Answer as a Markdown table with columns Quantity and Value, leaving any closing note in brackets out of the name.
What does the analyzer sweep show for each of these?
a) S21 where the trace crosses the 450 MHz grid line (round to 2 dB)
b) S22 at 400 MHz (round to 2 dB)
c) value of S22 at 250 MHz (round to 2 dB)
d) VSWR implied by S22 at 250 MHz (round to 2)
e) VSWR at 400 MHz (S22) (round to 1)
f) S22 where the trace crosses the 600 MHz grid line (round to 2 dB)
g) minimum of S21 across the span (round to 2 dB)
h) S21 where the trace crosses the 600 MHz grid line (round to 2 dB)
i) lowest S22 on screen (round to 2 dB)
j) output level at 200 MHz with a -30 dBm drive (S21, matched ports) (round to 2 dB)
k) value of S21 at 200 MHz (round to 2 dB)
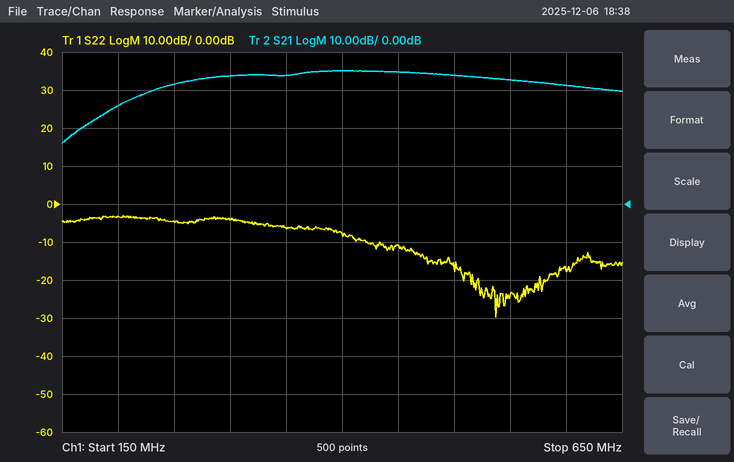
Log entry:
| Quantity | Value |
|---|---|
| S21 where the trace crosses the 450 MHz grid line | 34 dB |
| S22 at 400 MHz | -8 dB |
| value of S22 at 250 MHz | -4 dB |
| VSWR implied by S22 at 250 MHz | 4 |
| VSWR at 400 MHz (S22) | 2 |
| S22 where the trace crosses the 600 MHz grid line | -18 dB |
| minimum of S21 across the span | 16 dB |
| S21 where the trace crosses the 600 MHz grid line | 32 dB |
| lowest S22 on screen | -30 dB |
| output level at 200 MHz with a -30 dBm drive (S21, matched ports) | -4 dBm |
| value of S21 at 200 MHz | 26 dB |
